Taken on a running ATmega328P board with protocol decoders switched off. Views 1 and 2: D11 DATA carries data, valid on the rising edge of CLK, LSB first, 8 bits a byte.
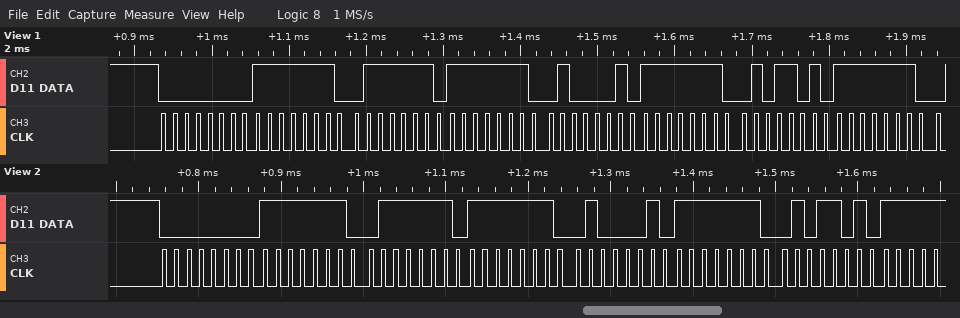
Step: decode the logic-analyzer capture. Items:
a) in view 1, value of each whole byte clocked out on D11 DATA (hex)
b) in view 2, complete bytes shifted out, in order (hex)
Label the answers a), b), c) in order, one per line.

a) 00 7F 7E 7F 42 7F 5A 7F
b) 00 7F 7E 7F 42 7F 5A
